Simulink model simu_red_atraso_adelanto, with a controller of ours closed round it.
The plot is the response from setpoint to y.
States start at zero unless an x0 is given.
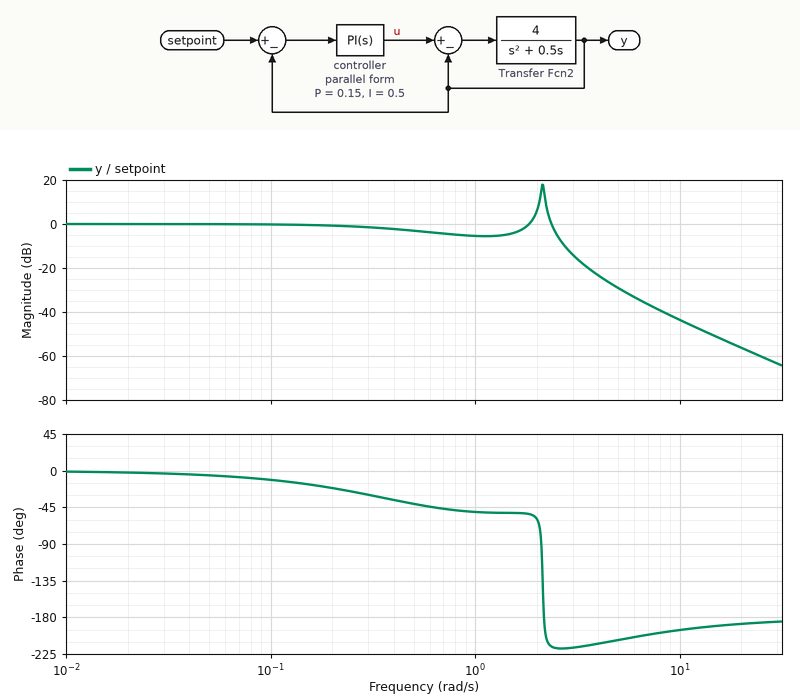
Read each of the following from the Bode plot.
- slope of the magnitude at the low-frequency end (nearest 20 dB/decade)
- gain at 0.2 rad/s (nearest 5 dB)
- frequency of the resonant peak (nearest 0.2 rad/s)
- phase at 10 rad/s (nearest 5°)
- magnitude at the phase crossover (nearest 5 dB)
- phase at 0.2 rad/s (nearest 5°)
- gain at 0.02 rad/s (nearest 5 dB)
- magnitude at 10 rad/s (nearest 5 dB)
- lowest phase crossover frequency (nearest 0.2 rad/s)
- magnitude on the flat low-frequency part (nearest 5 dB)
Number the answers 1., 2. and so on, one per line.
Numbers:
1. 0 dB/decade
2. 0 dB
3. 2.2 rad/s
4. -195°
5. 15 dB
6. -20°
7. 0 dB
8. -45 dB
9. 2.2 rad/s
10. 0 dB
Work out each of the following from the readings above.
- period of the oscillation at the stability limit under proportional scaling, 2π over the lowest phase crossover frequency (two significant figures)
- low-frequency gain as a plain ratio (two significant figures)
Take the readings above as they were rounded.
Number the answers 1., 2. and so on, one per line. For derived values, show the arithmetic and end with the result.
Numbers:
1. 2π / 2.2 = 2.9 s
2. 10^(0 / 20) = 1.0
